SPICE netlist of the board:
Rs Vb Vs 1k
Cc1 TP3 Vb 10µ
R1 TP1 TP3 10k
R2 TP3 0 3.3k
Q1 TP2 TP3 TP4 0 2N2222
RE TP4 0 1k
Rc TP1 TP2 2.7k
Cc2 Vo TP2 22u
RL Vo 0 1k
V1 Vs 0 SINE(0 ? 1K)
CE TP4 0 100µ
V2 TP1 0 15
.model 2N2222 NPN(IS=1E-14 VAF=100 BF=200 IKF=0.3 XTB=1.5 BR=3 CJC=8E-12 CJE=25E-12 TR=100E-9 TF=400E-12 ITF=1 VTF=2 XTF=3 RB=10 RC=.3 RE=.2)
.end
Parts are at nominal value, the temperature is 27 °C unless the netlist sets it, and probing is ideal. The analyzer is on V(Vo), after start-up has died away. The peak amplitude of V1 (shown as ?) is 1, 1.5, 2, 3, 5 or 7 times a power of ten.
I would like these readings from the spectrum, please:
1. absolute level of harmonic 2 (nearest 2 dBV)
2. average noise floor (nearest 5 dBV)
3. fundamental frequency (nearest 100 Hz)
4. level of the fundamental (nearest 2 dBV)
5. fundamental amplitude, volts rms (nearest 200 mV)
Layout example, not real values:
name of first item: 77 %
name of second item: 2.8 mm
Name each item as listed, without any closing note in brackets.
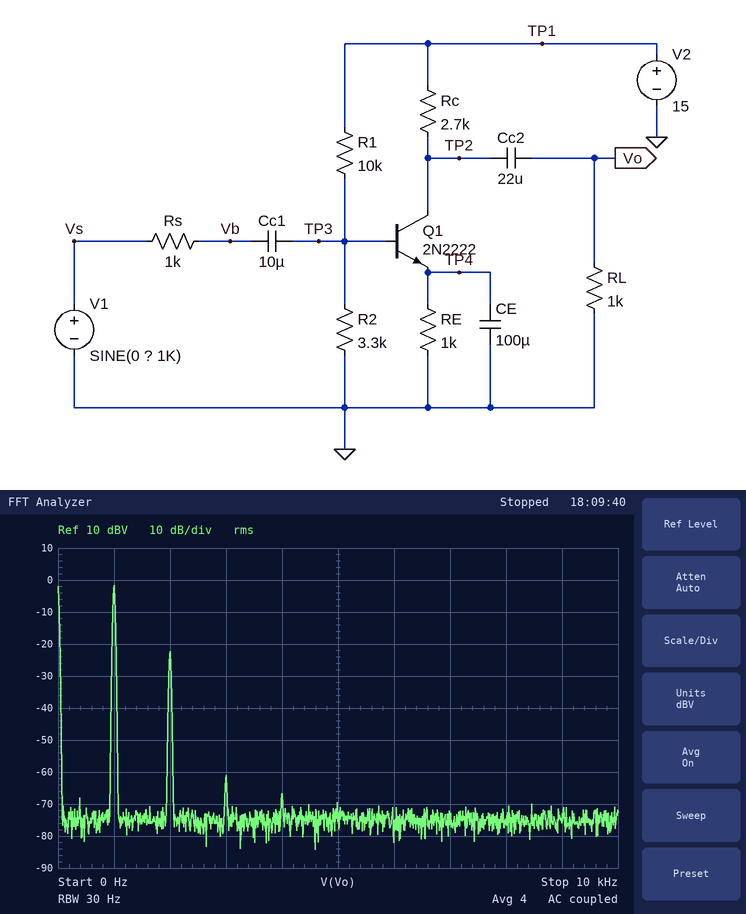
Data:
absolute level of harmonic 2: -22 dBV
average noise floor: -75 dBV
fundamental frequency: 1.0 kHz
level of the fundamental: -2 dBV
fundamental amplitude, volts rms: 800 mV
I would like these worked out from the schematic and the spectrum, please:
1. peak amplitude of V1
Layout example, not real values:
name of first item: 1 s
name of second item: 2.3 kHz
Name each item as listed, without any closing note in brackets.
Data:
peak amplitude of V1: 30 mV
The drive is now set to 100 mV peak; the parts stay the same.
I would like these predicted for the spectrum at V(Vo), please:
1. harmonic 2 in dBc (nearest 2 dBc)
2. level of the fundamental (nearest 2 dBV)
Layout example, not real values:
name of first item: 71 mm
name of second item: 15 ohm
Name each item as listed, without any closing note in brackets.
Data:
harmonic 2 in dBc: -10 dBc
level of the fundamental: 6 dBV
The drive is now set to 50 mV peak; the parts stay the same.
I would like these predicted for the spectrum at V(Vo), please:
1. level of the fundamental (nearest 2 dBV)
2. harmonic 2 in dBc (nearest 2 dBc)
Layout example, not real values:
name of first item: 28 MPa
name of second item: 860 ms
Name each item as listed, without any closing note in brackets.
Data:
level of the fundamental: 2 dBV
harmonic 2 in dBc: -16 dBc
